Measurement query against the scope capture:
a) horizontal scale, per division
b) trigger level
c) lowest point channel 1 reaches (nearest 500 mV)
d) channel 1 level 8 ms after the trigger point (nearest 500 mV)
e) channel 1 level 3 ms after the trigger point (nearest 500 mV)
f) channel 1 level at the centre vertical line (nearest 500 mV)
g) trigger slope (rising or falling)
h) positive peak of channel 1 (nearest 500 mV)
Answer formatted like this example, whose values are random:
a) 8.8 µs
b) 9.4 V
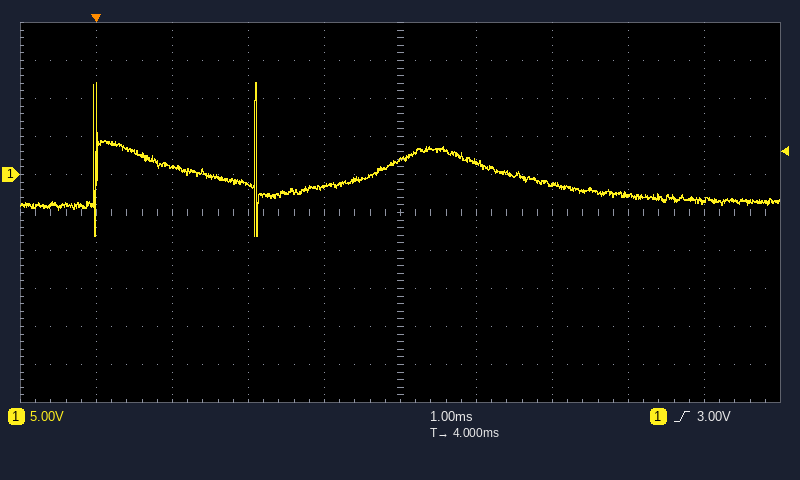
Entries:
a) 1 ms
b) 3.00 V
c) -8.0 V
d) -3.5 V
e) -1.5 V
f) 2.0 V
g) rising
h) 12.0 V
